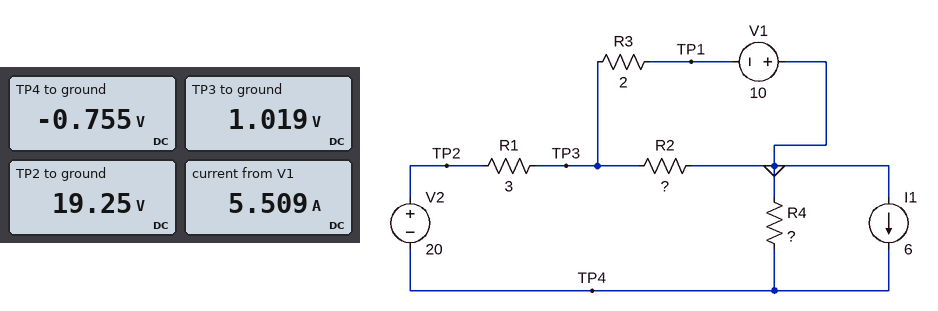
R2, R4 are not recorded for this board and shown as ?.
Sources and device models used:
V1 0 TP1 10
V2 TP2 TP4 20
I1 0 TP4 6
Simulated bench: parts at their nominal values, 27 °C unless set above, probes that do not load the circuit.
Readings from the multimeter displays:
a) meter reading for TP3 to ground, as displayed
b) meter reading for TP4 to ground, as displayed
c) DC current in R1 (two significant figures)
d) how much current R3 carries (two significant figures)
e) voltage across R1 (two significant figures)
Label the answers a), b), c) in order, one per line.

a) 1.019 V
b) -0.755 V
c) 6.1 A
d) 5.5 A
e) 18 V
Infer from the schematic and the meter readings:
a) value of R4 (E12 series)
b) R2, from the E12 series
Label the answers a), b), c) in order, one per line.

a) 10 Ω
b) 1.8 Ω
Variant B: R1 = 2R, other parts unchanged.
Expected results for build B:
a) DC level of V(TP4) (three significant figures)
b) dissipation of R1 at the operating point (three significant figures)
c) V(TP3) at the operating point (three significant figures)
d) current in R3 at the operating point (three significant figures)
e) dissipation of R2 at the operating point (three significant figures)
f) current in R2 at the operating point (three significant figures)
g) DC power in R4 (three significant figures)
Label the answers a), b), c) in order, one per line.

a) -5.45 V
b) 85.7 W
c) 1.46 V
d) 5.73 A
e) 1.19 W
f) 813 mA
g) 2.97 W
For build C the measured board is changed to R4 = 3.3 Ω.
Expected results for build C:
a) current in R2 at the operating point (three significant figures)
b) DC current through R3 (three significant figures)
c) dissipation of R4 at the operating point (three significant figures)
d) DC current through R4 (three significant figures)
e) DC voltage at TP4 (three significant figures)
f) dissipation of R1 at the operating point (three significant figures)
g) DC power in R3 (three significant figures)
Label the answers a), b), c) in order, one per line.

a) 603 mA
b) 5.54 A
c) 69.6 mW
d) 145 mA
e) -479 mV
f) 113 W
g) 61.4 W
